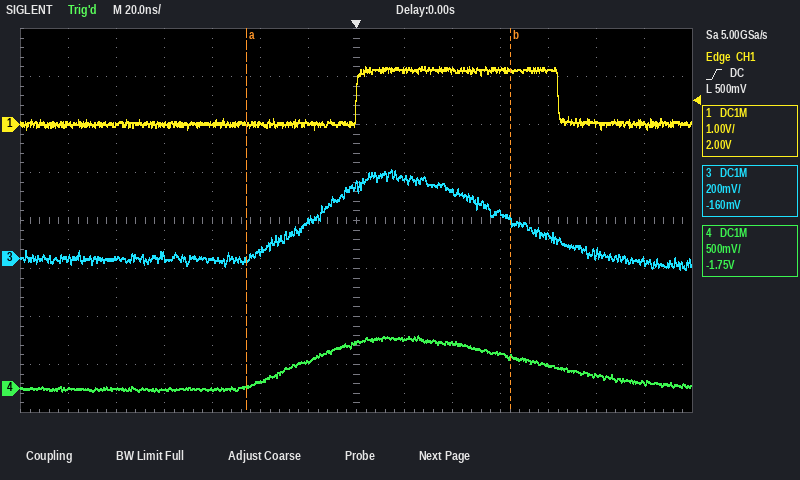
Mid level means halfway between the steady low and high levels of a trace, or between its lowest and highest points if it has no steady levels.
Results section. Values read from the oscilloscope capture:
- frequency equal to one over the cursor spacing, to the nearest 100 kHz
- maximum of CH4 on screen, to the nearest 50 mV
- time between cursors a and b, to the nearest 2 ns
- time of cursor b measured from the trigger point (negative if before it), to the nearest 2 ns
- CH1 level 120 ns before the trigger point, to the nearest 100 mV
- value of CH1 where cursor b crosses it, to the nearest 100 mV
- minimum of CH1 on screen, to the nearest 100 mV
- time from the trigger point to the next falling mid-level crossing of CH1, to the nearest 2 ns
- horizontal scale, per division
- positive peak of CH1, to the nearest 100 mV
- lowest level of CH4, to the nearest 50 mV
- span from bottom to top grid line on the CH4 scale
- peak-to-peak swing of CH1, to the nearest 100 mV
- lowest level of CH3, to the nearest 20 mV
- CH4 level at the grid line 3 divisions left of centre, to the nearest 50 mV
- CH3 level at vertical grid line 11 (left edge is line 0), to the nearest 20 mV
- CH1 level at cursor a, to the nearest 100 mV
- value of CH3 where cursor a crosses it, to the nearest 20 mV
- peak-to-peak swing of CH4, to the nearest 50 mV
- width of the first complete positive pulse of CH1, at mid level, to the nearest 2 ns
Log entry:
9.1 MHz
550 mV
110 ns
+64 ns
0.0 V
1.1 V
-100 mV
84 ns
20 ns
1.2 V
-50 mV
4 V
1.3 V
-40 mV
0 mV
100 mV
0.0 V
0 mV
600 mV
84 ns
